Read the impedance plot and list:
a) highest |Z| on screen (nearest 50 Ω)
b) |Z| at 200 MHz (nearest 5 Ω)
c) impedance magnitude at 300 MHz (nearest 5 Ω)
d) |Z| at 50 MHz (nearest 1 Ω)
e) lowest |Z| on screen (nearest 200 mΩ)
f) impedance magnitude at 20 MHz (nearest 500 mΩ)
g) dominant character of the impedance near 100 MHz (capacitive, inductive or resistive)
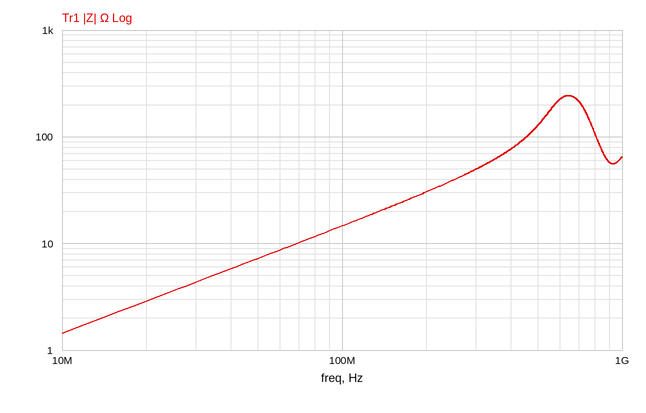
250 Ω
30 Ω
50 Ω
7 Ω
1.4 Ω
3.0 Ω
inductive
